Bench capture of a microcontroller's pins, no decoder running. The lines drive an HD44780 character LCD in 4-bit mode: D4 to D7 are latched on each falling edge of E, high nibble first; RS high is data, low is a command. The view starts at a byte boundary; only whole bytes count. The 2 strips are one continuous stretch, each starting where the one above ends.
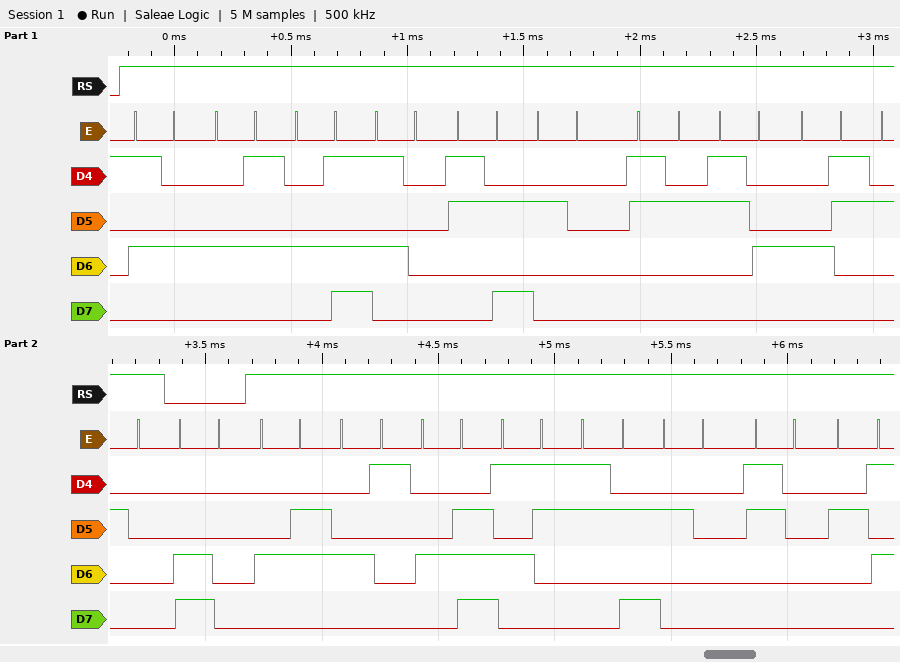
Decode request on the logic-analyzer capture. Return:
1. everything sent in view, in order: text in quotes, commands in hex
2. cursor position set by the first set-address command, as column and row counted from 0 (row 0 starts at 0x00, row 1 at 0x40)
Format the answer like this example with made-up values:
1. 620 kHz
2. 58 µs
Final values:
1. "TEMP: 24C " 0xC0 "FANS: 0%"
2. column 0, row 1
